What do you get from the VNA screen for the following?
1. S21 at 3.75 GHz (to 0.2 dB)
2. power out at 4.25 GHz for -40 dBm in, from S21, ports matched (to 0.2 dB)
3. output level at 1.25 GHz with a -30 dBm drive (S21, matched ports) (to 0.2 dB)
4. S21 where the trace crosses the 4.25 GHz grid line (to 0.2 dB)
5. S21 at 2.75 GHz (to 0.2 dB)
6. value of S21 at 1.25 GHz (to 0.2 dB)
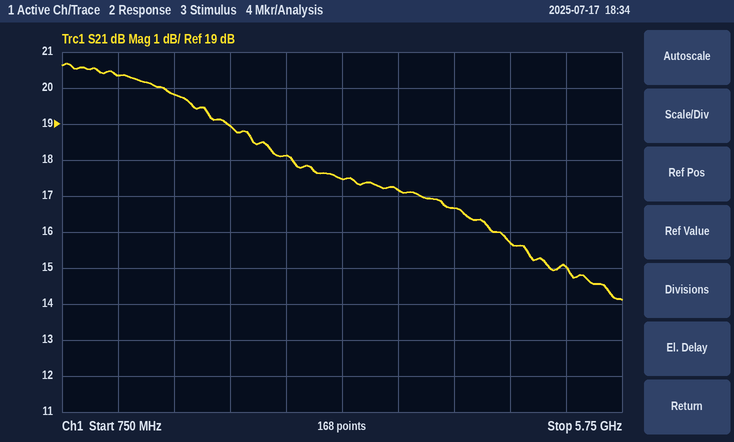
17.2 dB
-23.4 dBm
-9.6 dBm
16.6 dB
18.2 dB
20.4 dB
